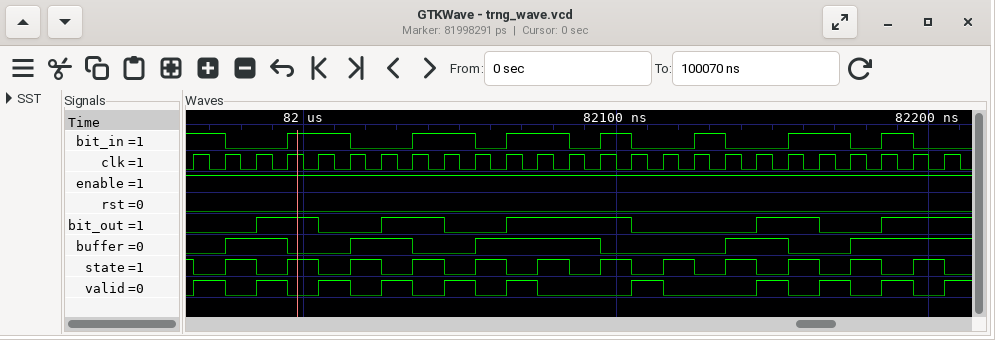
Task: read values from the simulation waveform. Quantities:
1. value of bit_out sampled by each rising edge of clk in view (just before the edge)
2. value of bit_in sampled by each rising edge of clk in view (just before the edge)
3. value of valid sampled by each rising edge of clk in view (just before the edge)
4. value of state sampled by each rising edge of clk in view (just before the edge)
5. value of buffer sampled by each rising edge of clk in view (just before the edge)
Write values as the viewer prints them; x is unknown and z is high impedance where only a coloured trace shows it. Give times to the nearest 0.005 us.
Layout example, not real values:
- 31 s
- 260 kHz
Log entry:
- 0 0 0 1 1 0 0 1 1 0 0 1 1 1 1 0 0 0 0 1 1 0 0 1 1
- 1 1 0 0 1 1 0 0 1 1 0 1 1 0 1 0 0 1 0 0 1 1 0 1 0
- 0 1 0 1 0 1 0 1 0 1 0 1 0 0 0 1 0 0 0 1 0 1 0 1 0
- 1 0 1 0 1 0 1 0 1 0 1 0 1 0 1 0 1 0 1 0 1 0 1 0 1
- 0 0 1 1 0 0 1 1 0 0 1 1 1 1 0 0 0 0 1 1 0 0 1 1 1
